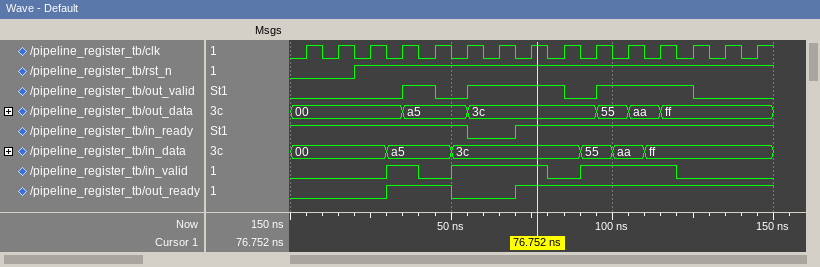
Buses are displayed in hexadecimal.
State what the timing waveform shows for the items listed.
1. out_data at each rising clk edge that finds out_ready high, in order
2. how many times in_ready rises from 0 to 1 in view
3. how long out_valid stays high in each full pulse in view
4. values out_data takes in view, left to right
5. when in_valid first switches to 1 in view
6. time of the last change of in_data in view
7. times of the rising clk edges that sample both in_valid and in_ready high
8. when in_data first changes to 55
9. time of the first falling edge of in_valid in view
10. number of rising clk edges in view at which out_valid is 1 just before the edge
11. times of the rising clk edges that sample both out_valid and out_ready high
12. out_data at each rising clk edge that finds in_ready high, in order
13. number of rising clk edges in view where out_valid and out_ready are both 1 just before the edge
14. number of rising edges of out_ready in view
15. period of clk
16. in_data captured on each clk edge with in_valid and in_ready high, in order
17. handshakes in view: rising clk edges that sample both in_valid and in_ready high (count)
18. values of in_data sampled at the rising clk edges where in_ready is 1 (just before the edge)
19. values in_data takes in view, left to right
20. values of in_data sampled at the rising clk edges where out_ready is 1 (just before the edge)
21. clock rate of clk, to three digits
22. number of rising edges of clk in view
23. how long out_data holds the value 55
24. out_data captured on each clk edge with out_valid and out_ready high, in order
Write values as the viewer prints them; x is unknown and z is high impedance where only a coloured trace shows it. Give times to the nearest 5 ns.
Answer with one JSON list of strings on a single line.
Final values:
["00, a5, 3c, 3c, 3c, 55, aa, ff, ff, ff", "1", "10 ns, 30 ns, 30 ns", "00, a5, 3c, 55, aa, ff", "30 ns", "110 ns", "35 ns, 55 ns, 75 ns, 95 ns, 105 ns, 115 ns", "90 ns", "40 ns", "7", "45 ns, 75 ns, 85 ns, 105 ns, 115 ns, 125 ns", "00, 00, 00, 00, a5, a5, 3c, 3c, 3c, 55, aa, ff, ff, ff", "6", "2", "10 ns", "a5, 3c, 3c, 55, aa, ff", "6", "00, 00, 00, a5, a5, 3c, 3c, 3c, 55, aa, ff, ff, ff, ff", "00, a5, 3c, 55, aa, ff", "a5, a5, 3c, 3c, 55, aa, ff, ff, ff, ff", "100 MHz", "15", "10 ns", "a5, 3c, 3c, 55, aa, ff"]
